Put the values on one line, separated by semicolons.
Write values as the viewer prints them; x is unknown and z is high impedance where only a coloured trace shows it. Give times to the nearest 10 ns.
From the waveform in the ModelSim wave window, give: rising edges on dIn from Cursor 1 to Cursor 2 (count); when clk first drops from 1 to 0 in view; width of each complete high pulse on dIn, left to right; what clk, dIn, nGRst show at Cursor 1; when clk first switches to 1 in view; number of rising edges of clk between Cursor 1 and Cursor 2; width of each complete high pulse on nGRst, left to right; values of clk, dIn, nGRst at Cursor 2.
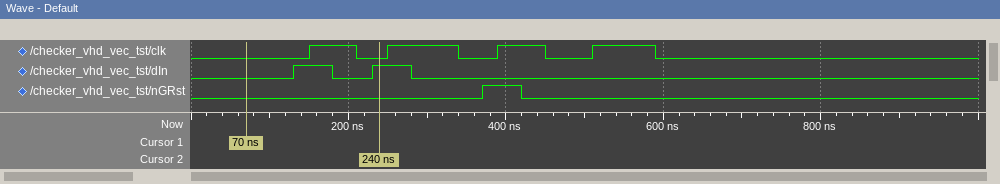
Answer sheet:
2; 210 ns; 50 ns, 50 ns; clk=0, dIn=0, nGRst=0; 150 ns; 1; 50 ns; clk=0, dIn=1, nGRst=0
